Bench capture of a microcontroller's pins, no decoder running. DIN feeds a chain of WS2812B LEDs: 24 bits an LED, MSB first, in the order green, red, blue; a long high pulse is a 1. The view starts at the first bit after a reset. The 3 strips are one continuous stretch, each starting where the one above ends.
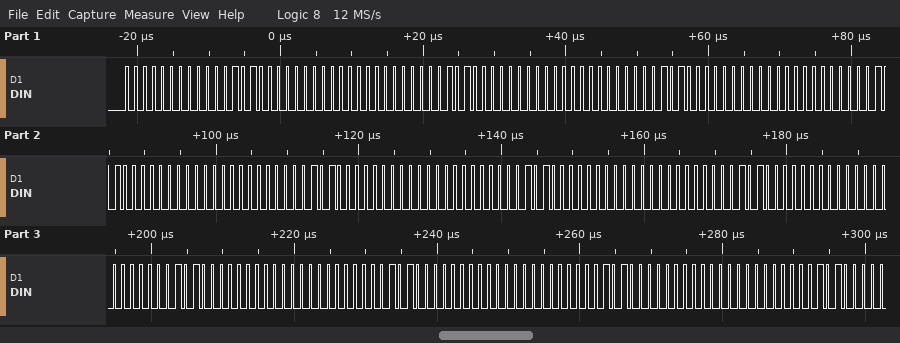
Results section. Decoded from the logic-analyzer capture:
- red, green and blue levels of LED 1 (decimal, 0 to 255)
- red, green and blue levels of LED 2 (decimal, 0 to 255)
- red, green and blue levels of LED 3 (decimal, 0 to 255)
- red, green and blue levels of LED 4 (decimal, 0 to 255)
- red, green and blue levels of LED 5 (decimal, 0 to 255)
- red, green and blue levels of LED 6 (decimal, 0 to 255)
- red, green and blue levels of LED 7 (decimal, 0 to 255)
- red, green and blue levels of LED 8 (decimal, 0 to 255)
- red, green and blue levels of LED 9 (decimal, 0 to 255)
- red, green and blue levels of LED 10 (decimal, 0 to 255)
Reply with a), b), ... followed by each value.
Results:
a) 10, 0, 0
b) 10, 0, 0
c) 10, 0, 0
d) 10, 0, 0
e) 10, 0, 0
f) 10, 0, 0
g) 10, 0, 0
h) 10, 0, 0
i) 10, 0, 0
j) 10, 0, 0
